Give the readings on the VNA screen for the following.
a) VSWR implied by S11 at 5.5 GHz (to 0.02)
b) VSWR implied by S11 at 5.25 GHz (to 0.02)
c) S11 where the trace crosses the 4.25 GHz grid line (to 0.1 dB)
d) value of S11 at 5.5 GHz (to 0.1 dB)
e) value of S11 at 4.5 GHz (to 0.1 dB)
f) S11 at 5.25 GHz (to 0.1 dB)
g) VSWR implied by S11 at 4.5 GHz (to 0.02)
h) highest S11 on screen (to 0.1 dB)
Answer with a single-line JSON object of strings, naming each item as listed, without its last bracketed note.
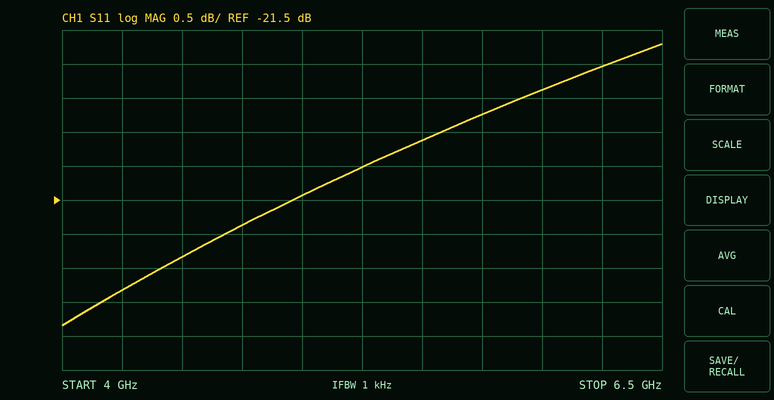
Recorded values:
{"VSWR implied by S11 at 5.5 GHz": "1.20", "VSWR implied by S11 at 5.25 GHz": "1.20", "S11 where the trace crosses the 4.25 GHz grid line": "-22.8 dB", "value of S11 at 5.5 GHz": "-20.6 dB", "value of S11 at 4.5 GHz": "-22.3 dB", "S11 at 5.25 GHz": "-21.0 dB", "VSWR implied by S11 at 4.5 GHz": "1.16", "highest S11 on screen": "-19.2 dB"}
